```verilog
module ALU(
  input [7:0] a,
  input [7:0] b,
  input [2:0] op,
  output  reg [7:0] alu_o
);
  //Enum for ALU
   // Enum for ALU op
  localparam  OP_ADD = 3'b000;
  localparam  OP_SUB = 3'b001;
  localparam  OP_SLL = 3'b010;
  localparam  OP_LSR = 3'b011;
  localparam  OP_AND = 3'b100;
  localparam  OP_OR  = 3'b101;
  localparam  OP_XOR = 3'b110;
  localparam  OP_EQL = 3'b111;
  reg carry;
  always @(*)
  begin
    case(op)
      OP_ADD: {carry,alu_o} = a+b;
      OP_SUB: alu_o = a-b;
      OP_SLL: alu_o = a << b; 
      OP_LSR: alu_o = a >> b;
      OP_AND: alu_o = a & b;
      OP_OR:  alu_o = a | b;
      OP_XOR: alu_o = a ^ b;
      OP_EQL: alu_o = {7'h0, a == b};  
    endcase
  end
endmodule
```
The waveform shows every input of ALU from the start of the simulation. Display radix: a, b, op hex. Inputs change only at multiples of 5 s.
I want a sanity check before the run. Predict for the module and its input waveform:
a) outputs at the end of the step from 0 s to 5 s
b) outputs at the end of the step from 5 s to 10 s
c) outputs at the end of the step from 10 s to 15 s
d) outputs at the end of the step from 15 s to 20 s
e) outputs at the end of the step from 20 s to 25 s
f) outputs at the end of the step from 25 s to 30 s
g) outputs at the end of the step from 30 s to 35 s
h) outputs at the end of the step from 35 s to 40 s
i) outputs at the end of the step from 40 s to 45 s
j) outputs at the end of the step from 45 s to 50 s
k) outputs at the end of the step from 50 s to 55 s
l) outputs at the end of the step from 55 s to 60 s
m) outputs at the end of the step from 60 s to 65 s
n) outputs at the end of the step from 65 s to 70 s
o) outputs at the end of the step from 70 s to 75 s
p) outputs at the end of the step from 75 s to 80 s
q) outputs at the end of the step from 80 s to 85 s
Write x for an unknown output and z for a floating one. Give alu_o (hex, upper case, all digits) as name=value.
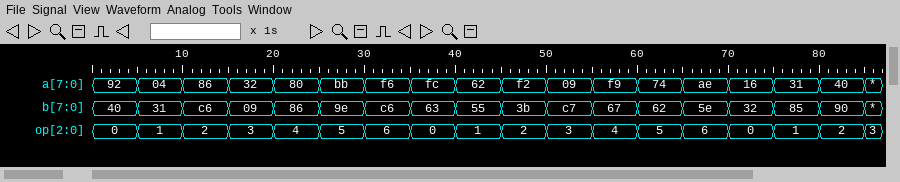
alu_o=D2
alu_o=D3
alu_o=00
alu_o=00
alu_o=80
alu_o=BF
alu_o=30
alu_o=5F
alu_o=0D
alu_o=00
alu_o=00
alu_o=61
alu_o=76
alu_o=F0
alu_o=48
alu_o=AC
alu_o=00
